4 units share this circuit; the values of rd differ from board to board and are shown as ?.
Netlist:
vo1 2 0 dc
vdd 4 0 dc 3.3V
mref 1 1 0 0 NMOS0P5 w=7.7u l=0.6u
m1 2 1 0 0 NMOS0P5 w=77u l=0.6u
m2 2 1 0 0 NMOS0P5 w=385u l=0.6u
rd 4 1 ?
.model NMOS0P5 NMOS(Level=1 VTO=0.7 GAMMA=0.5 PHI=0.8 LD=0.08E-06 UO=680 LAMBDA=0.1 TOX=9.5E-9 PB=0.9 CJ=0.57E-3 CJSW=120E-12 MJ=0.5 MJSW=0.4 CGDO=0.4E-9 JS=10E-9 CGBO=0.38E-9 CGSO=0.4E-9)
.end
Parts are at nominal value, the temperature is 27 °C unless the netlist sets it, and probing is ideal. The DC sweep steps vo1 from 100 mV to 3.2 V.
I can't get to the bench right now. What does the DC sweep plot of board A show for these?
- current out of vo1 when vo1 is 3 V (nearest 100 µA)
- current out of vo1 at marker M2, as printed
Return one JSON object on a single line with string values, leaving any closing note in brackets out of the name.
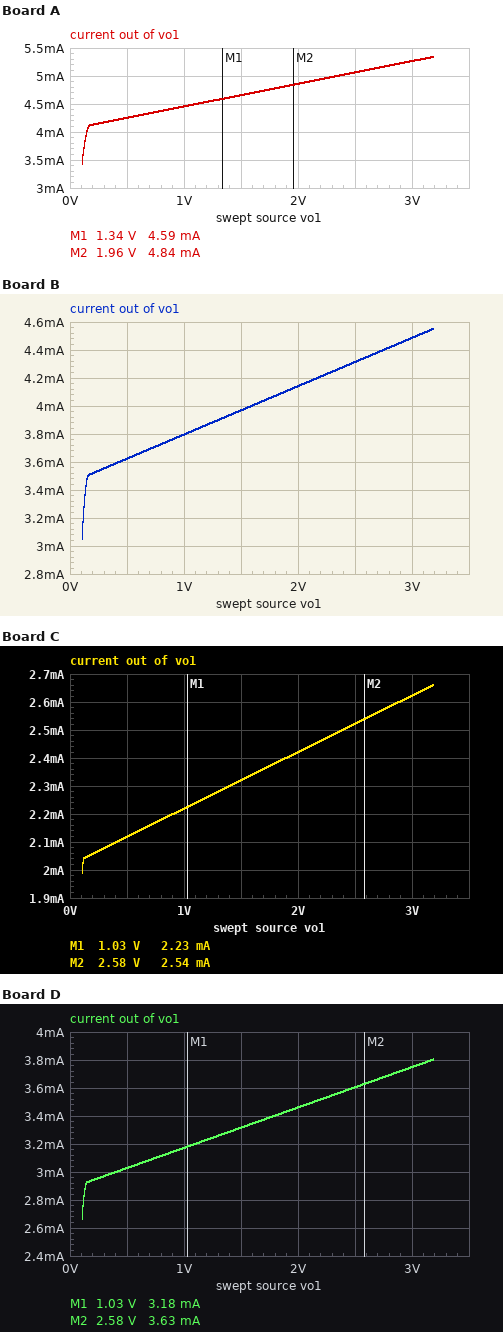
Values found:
{"current out of vo1 when vo1 is 3 V": "5.3 mA", "current out of vo1 at marker M2, as printed": "4.84 mA"}
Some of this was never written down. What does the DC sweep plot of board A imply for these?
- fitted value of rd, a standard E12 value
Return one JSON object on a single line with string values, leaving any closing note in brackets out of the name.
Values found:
{"fitted value of rd, a standard E12 value": "33 kΩ"}
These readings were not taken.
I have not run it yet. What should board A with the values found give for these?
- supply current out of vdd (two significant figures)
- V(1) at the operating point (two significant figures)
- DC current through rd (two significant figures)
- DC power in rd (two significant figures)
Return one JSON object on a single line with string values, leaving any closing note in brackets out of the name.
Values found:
{"supply current out of vdd": "73 µA", "V(1) at the operating point": "880 mV", "DC current through rd": "73 µA", "DC power in rd": "180 µW"}
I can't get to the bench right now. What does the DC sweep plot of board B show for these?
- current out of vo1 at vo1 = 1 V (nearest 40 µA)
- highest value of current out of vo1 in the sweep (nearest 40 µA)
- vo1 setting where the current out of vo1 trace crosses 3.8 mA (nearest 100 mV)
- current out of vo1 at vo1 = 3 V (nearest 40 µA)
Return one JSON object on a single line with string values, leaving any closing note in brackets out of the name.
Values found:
{"current out of vo1 at vo1 = 1 V": "3.80 mA", "highest value of current out of vo1 in the sweep": "4.56 mA", "vo1 setting where the current out of vo1 trace crosses 3.8 mA": "1.0 V", "current out of vo1 at vo1 = 3 V": "4.48 mA"}
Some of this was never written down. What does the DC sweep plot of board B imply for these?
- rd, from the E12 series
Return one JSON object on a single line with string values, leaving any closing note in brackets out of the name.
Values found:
{"rd, from the E12 series": "39 kΩ"}
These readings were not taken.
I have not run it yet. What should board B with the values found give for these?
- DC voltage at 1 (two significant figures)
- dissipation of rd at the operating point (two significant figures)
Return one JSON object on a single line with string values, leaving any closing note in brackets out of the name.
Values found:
{"DC voltage at 1": "860 mV", "dissipation of rd at the operating point": "150 µW"}
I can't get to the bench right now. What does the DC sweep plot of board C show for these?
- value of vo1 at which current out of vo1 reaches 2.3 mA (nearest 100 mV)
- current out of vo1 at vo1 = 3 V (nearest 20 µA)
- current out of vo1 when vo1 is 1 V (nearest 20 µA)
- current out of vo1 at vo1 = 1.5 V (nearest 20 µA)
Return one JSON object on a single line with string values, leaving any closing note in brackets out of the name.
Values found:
{"value of vo1 at which current out of vo1 reaches 2.3 mA": "1.4 V", "current out of vo1 at vo1 = 3 V": "2.62 mA", "current out of vo1 when vo1 is 1 V": "2.22 mA", "current out of vo1 at vo1 = 1.5 V": "2.32 mA"}
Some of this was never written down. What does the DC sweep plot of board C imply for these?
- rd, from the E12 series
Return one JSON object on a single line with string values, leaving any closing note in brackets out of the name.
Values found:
{"rd, from the E12 series": "68 kΩ"}
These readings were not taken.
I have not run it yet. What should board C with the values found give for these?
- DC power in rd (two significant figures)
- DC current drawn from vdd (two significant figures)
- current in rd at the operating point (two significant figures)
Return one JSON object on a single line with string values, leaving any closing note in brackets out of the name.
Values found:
{"DC power in rd": "90 µW", "DC current drawn from vdd": "36 µA", "current in rd at the operating point": "36 µA"}
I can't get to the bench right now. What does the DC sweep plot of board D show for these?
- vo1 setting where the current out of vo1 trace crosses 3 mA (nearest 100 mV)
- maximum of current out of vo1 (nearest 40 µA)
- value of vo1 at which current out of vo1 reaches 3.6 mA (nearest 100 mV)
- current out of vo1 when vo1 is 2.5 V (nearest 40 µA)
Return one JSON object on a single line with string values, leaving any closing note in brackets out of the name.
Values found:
{"vo1 setting where the current out of vo1 trace crosses 3 mA": "400 mV", "maximum of current out of vo1": "3.80 mA", "value of vo1 at which current out of vo1 reaches 3.6 mA": "2.5 V", "current out of vo1 when vo1 is 2.5 V": "3.60 mA"}
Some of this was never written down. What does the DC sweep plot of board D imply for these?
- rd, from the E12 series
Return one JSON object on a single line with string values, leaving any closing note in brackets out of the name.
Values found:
{"rd, from the E12 series": "47 kΩ"}
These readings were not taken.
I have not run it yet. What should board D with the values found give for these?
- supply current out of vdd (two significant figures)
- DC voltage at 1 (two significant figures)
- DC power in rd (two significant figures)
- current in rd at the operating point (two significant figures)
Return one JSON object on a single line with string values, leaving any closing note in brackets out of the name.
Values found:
{"supply current out of vdd": "52 µA", "DC voltage at 1": "850 mV", "DC power in rd": "130 µW", "current in rd at the operating point": "52 µA"}
